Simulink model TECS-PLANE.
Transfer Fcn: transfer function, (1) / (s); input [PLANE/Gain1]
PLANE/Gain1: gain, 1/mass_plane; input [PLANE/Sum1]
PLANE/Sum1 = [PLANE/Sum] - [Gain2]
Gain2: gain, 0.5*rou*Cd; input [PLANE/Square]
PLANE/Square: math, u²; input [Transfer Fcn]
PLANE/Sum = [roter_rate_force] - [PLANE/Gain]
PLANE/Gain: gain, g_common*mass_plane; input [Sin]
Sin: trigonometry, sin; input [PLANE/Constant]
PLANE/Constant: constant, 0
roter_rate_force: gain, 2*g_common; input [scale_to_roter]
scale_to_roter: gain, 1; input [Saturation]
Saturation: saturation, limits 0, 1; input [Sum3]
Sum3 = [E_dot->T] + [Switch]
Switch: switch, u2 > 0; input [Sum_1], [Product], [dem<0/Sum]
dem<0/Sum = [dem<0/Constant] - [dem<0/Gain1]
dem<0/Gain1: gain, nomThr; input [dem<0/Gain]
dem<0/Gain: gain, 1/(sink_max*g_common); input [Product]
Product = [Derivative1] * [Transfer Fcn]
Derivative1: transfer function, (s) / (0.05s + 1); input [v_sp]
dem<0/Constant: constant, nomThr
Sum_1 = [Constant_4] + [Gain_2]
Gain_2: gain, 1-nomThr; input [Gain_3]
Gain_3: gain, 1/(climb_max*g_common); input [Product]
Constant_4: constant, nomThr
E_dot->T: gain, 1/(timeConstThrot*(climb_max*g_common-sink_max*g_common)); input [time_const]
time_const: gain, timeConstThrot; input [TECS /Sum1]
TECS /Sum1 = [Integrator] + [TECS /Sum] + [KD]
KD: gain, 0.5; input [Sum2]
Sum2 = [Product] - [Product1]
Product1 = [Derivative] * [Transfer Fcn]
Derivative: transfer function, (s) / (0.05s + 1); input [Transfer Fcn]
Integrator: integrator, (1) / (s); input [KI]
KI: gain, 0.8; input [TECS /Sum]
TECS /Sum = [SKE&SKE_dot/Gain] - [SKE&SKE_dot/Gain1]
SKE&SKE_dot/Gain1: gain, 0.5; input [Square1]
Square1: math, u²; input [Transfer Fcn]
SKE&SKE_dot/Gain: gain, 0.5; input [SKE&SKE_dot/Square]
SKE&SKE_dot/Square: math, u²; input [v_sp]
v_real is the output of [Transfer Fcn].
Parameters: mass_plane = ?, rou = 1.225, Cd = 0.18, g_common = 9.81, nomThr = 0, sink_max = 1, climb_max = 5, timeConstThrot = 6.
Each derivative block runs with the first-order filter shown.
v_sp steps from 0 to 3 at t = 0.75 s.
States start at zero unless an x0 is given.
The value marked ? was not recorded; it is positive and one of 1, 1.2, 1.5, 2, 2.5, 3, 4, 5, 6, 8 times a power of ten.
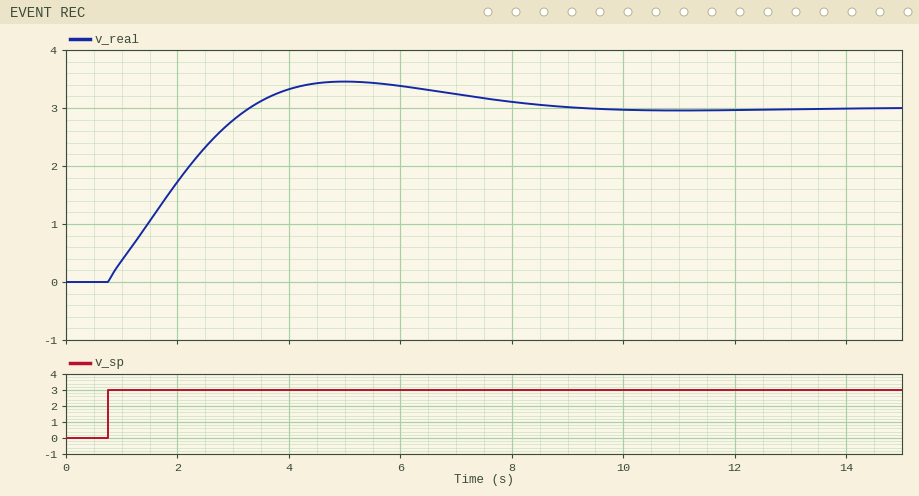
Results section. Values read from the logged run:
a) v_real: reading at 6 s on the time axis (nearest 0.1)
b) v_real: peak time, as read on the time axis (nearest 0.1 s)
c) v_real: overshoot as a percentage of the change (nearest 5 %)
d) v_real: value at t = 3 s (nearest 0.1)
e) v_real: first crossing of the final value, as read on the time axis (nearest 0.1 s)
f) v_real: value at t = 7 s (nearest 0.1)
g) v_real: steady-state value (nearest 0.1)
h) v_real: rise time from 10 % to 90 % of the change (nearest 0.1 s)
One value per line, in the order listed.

3.4
5.0 s
15 %
2.8
3.3 s
3.2
3.0
1.9 s
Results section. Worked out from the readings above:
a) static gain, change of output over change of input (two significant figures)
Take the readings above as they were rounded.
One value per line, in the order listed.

1.0
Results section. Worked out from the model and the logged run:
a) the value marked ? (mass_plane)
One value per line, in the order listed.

2
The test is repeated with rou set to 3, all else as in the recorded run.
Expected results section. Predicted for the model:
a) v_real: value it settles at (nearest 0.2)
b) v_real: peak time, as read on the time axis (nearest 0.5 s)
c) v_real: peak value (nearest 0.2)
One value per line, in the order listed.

3.0
5.5 s
3.2
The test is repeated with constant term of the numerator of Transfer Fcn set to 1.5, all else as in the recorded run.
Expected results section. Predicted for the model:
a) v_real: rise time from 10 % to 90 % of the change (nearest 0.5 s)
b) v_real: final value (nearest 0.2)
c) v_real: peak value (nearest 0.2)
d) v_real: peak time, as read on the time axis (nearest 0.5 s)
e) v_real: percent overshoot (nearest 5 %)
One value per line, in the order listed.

1.5 s
3.0
3.4
4.5 s
10 %
